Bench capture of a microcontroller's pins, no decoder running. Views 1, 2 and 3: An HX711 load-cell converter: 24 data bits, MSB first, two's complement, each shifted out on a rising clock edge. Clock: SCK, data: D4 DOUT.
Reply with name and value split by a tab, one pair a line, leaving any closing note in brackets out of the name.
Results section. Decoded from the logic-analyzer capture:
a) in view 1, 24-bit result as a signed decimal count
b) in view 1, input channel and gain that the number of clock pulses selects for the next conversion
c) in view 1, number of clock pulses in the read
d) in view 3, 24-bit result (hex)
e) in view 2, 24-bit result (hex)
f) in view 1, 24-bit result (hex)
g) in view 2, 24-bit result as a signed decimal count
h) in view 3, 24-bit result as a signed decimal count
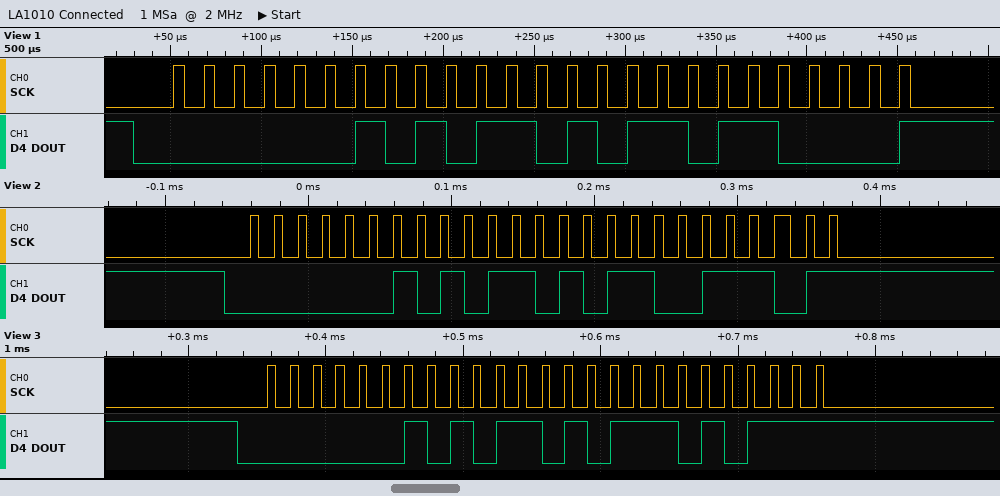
in view 1, 24-bit result as a signed decimal count	177584
in view 1, input channel and gain that the number of clock pulses selects for the next conversion	channel A, gain 128
in view 1, number of clock pulses in the read	25
in view 3, 24-bit result	0x02B5D7
in view 2, 24-bit result	0x02B59D
in view 1, 24-bit result	0x02B5B0
in view 2, 24-bit result as a signed decimal count	177565
in view 3, 24-bit result as a signed decimal count	177623
